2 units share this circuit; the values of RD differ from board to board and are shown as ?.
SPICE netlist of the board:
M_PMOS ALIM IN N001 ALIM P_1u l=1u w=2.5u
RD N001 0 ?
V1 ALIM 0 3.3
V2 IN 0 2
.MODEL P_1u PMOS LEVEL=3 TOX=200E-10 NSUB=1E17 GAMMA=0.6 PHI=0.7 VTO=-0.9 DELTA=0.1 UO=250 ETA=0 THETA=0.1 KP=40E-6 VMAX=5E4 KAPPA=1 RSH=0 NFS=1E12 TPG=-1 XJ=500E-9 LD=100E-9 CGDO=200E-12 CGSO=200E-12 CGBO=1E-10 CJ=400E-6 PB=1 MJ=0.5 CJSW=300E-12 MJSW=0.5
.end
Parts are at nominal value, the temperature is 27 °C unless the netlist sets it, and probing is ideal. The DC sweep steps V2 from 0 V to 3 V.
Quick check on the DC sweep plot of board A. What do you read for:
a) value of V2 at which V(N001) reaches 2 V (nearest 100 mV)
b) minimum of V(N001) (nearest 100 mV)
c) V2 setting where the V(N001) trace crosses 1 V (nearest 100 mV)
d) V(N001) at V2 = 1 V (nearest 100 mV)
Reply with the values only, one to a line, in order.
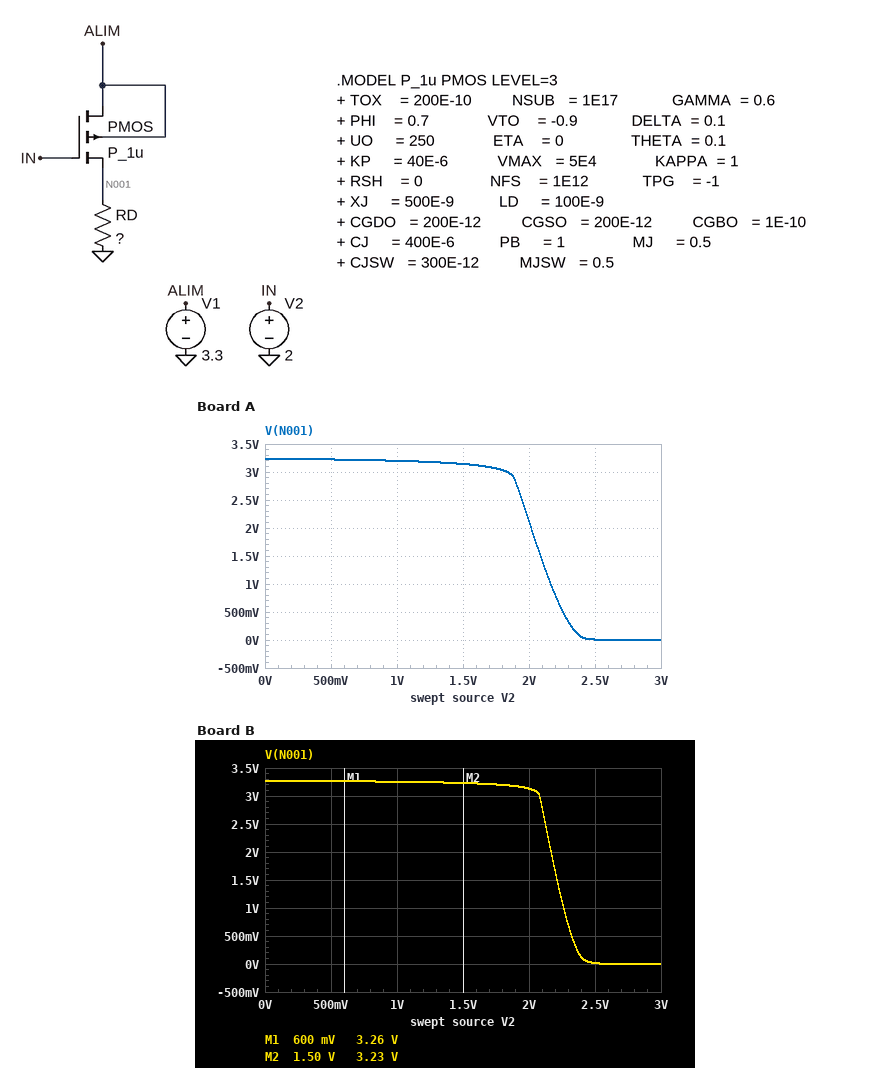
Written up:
2.0 V
0 V
2.2 V
3.2 V
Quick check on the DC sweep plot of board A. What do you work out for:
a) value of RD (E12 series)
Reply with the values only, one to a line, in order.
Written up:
220 kΩ
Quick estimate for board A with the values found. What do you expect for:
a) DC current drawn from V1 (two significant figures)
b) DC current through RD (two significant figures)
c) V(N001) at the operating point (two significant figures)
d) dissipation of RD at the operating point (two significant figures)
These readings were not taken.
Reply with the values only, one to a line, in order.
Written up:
9.6 µA
9.6 µA
2.1 V
20 µW
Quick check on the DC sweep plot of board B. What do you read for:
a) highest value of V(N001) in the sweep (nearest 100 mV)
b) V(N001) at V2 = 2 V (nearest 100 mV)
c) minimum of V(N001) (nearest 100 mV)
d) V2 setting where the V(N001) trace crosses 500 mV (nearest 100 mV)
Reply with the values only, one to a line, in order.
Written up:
3.3 V
3.1 V
0 V
2.3 V
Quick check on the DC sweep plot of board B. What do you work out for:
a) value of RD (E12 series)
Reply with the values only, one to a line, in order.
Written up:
470 kΩ
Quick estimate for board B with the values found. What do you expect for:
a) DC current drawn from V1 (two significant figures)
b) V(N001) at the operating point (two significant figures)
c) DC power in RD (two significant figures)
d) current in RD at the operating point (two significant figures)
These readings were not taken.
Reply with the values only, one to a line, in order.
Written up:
6.7 µA
3.1 V
21 µW
6.7 µA
